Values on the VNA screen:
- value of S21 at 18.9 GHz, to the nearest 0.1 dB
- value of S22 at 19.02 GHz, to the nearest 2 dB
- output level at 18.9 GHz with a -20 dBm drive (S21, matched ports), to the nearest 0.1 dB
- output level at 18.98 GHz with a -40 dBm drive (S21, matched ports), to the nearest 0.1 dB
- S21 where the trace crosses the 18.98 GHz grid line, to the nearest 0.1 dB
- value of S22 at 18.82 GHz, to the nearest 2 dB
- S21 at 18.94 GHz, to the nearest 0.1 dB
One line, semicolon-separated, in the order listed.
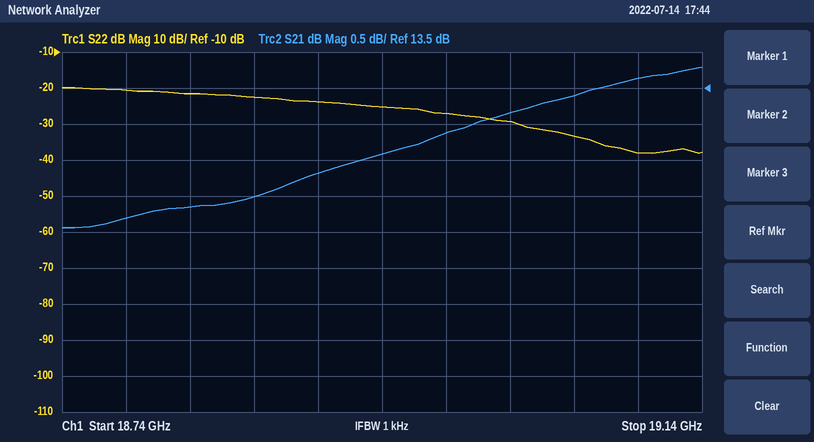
12.3 dB; -30 dB; -7.7 dBm; -27.1 dBm; 12.9 dB; -22 dB; 12.6 dB
